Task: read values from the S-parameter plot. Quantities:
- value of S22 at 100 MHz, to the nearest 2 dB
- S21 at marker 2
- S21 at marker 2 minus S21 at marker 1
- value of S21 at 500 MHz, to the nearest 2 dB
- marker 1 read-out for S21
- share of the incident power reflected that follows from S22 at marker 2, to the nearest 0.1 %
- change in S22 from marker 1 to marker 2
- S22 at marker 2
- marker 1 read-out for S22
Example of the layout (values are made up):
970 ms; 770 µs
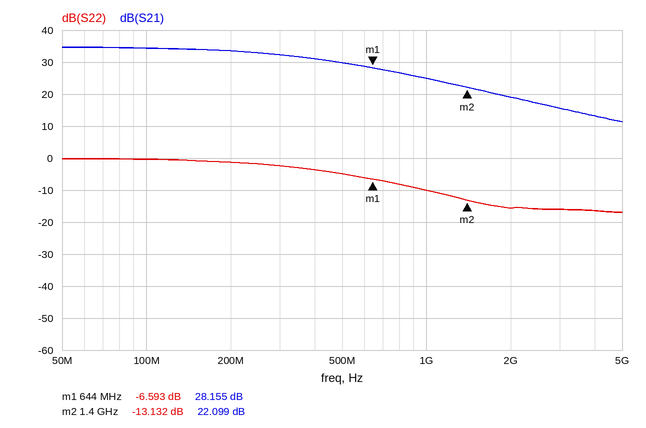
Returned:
0 dB; 22.099 dB; -6.056 dB; 30 dB; 28.155 dB; 4.9 %; -6.539 dB; -13.132 dB; -6.593 dB
